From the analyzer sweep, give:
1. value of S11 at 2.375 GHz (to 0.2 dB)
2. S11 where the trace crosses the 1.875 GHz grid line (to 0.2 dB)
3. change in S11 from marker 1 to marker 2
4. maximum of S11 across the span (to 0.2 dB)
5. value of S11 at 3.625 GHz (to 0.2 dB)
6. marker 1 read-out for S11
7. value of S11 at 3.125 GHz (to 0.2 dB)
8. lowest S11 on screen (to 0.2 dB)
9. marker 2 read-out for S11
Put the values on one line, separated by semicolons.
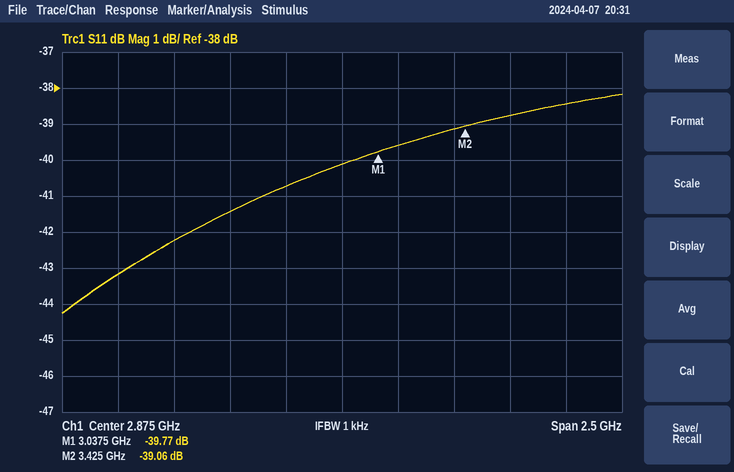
-41.4 dB; -43.2 dB; 0.71 dB; -38.2 dB; -38.8 dB; -39.77 dB; -39.6 dB; -44.2 dB; -39.06 dB
